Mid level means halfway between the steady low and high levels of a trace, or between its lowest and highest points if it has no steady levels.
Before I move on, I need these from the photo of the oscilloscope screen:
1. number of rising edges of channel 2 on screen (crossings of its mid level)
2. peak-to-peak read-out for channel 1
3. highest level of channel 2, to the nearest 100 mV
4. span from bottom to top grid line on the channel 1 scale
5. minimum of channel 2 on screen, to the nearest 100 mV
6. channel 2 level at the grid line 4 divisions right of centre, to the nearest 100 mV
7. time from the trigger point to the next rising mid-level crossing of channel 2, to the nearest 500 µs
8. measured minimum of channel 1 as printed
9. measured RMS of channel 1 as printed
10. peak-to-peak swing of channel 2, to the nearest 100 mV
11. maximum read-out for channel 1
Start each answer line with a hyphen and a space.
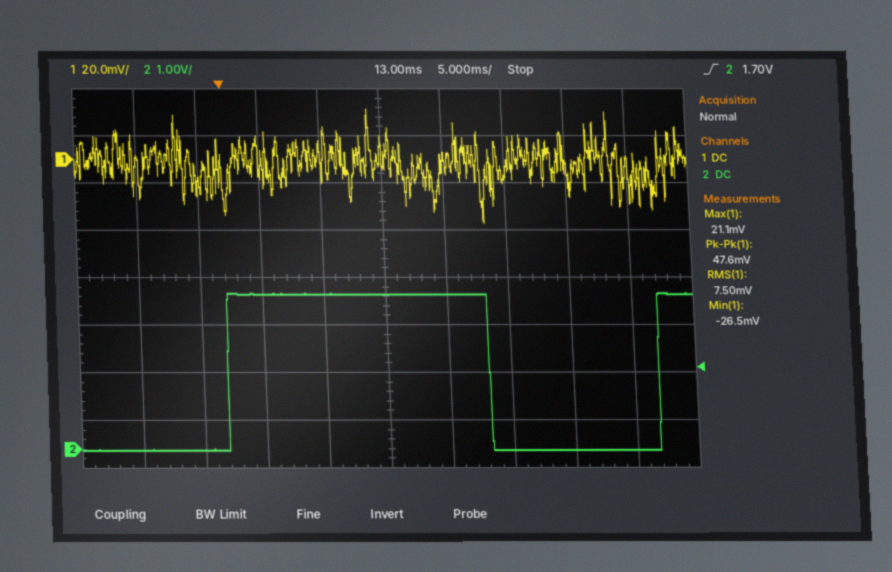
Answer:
- 2
- 47.6 mV
- 3.3 V
- 160 mV
- 0.0 V
- 0.0 V
- 35.0 ms
- -26.5 mV
- 7.50 mV
- 3.3 V
- 21.1 mV
